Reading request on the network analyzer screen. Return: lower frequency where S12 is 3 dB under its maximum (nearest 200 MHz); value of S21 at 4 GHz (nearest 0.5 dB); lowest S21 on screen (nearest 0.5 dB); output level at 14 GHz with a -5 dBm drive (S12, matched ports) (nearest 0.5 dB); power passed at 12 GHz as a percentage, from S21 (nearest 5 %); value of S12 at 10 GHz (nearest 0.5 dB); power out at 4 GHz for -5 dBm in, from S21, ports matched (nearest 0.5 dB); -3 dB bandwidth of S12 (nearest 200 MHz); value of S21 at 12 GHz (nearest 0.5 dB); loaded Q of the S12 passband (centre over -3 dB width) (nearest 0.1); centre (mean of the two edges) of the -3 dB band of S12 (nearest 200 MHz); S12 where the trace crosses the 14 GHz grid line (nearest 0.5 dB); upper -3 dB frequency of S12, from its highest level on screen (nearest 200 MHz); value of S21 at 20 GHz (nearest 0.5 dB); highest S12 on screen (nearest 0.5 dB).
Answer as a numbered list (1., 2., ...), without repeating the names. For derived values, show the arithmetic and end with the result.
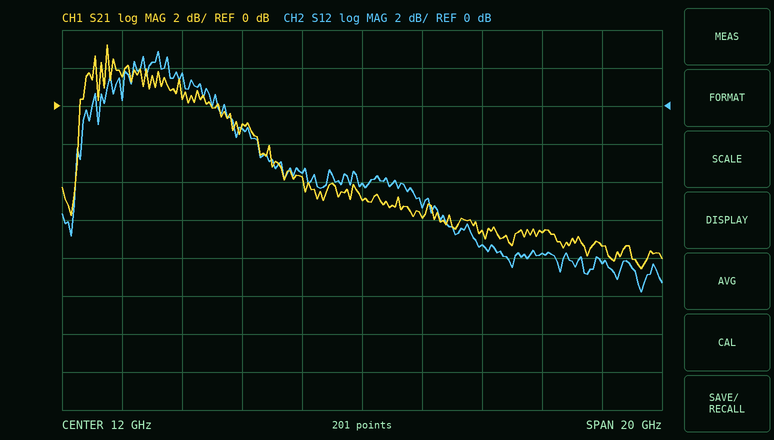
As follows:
1. 3.2 GHz
2. 1.5 dB
3. -8.5 dB
4. -5 dBm + (-5.5 dB) = -10.5 dBm
5. 10^(-5/10) ≈ 31.6 %, so 30 % to the nearest 5 %
6. -3.5 dB
7. -5 dBm + (1.5 dB) = -3.5 dBm
8. 7.2 GHz − 3.2 GHz = 4.0 GHz
9. -5.0 dB
10. 5.2 GHz / 4 GHz ≈ 1.3
11. 5.2 GHz
12. -5.5 dB
13. 7.2 GHz
14. -7.5 dB
15. 3.0 dB
